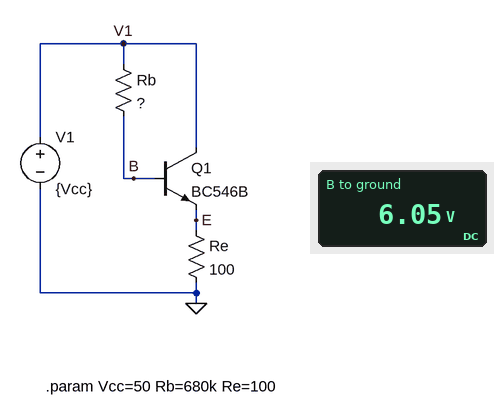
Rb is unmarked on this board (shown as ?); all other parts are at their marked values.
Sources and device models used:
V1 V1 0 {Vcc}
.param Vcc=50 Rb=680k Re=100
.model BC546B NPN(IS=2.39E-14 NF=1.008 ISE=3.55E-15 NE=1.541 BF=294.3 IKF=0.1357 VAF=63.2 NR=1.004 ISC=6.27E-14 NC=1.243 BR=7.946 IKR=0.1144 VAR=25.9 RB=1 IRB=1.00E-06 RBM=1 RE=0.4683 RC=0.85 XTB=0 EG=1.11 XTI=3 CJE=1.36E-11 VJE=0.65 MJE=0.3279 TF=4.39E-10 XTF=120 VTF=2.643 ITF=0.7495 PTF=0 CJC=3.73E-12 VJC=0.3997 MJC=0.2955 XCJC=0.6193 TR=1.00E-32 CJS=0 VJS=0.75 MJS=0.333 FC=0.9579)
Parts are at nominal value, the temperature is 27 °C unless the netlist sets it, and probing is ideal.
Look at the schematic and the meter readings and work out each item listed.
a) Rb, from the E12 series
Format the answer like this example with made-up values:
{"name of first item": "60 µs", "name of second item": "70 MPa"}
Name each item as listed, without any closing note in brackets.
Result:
{"Rb, from the E12 series": "330 kΩ"}
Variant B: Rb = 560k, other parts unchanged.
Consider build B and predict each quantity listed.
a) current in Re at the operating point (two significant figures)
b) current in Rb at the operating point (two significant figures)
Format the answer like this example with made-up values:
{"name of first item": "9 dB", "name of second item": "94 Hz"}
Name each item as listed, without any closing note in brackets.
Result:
{"current in Re at the operating point": "35 mA", "current in Rb at the operating point": "82 µA"}
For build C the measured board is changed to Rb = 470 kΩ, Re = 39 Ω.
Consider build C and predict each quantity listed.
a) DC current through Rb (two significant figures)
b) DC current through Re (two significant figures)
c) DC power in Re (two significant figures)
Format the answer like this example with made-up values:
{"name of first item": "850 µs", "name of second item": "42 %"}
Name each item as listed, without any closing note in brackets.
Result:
{"DC current through Rb": "100 µA", "DC current through Re": "43 mA", "DC power in Re": "73 mW"}
